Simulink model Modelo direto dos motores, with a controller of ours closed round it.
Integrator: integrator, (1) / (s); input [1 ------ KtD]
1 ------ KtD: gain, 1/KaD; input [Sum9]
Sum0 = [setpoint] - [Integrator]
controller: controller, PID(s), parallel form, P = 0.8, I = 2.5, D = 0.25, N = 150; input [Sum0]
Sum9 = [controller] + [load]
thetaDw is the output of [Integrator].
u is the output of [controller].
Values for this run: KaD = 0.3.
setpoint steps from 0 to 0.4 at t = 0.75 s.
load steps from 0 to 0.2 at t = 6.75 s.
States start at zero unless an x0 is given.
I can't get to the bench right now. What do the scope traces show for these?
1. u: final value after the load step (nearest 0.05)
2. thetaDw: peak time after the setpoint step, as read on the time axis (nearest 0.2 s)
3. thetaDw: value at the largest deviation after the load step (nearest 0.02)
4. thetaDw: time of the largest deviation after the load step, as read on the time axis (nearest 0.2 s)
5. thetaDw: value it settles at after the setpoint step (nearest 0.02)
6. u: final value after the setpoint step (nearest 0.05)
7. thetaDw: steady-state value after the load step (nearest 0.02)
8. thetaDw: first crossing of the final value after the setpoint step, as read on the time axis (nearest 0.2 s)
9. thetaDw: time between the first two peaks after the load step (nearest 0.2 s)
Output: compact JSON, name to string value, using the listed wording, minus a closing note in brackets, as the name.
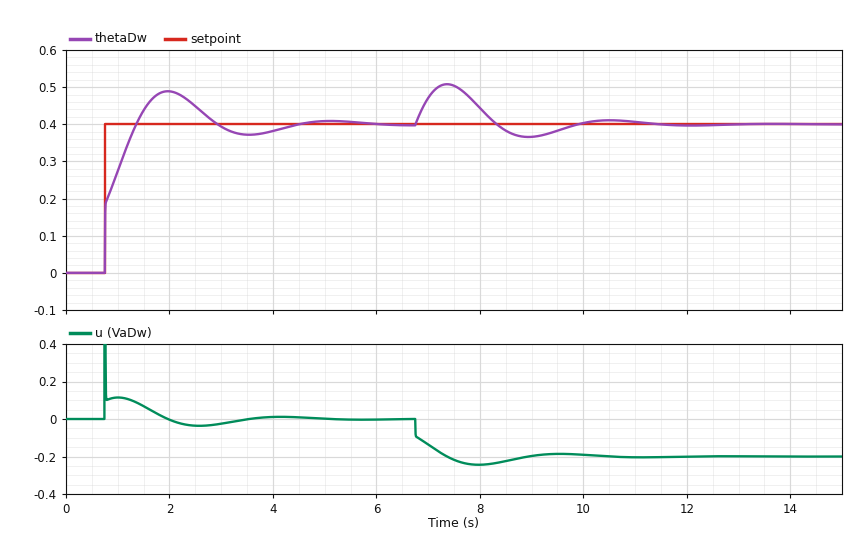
{"u: final value after the load step": "-0.20", "thetaDw: peak time after the setpoint step, as read on the time axis": "2.0 s", "thetaDw: value at the largest deviation after the load step": "0.50", "thetaDw: time of the largest deviation after the load step, as read on the time axis": "7.4 s", "thetaDw: value it settles at after the setpoint step": "0.40", "u: final value after the setpoint step": "0.00", "thetaDw: steady-state value after the load step": "0.40", "thetaDw: first crossing of the final value after the setpoint step, as read on the time axis": "1.4 s", "thetaDw: time between the first two peaks after the load step": "3.2 s"}
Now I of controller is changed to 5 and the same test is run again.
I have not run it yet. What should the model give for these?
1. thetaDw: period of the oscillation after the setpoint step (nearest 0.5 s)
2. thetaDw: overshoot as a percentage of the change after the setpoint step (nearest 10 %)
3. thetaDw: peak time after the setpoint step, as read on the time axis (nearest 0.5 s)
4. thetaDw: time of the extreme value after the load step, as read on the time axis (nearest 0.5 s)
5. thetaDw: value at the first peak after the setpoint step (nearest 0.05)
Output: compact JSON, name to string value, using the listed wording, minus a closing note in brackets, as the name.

{"thetaDw: period of the oscillation after the setpoint step": "2.0 s", "thetaDw: overshoot as a percentage of the change after the setpoint step": "30 %", "thetaDw: peak time after the setpoint step, as read on the time axis": "1.5 s", "thetaDw: time of the extreme value after the load step, as read on the time axis": "7.0 s", "thetaDw: value at the first peak after the setpoint step": "0.50"}
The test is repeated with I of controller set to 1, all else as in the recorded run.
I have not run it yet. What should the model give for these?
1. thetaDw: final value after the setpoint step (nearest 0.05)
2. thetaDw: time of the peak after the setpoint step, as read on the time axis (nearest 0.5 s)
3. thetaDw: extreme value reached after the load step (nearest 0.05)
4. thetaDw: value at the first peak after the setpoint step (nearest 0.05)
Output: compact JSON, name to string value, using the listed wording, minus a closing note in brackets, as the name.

{"thetaDw: final value after the setpoint step": "0.40", "thetaDw: time of the peak after the setpoint step, as read on the time axis": "2.5 s", "thetaDw: extreme value reached after the load step": "0.55", "thetaDw: value at the first peak after the setpoint step": "0.45"}
